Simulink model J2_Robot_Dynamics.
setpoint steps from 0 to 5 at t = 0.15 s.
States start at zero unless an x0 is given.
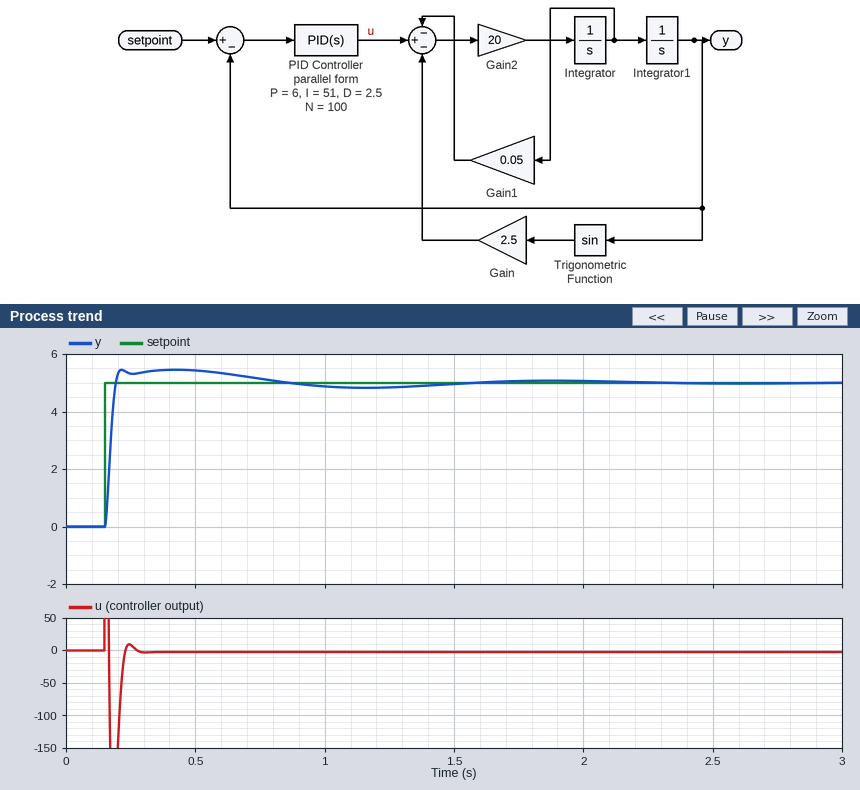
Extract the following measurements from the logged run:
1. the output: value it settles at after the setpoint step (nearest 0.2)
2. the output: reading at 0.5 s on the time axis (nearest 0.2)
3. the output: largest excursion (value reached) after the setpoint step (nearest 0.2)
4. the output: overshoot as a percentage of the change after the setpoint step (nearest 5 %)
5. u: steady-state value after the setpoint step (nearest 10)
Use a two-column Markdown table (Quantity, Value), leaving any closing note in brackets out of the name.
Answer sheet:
| Quantity | Value |
|---|---|
| the output: value it settles at after the setpoint step | 5.0 |
| the output: reading at 0.5 s on the time axis | 5.4 |
| the output: largest excursion (value reached) after the setpoint step | 5.4 |
| the output: overshoot as a percentage of the change after the setpoint step | 10 % |
| u: steady-state value after the setpoint step | 0 |
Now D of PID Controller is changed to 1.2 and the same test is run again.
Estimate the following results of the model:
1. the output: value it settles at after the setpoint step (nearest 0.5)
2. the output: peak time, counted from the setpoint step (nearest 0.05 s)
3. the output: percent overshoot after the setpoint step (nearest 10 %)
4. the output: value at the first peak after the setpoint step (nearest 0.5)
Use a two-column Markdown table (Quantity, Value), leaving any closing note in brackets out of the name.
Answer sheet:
| Quantity | Value |
|---|---|
| the output: value it settles at after the setpoint step | 5.0 |
| the output: peak time, counted from the setpoint step | 0.20 s |
| the output: percent overshoot after the setpoint step | 20 % |
| the output: value at the first peak after the setpoint step | 6.0 |
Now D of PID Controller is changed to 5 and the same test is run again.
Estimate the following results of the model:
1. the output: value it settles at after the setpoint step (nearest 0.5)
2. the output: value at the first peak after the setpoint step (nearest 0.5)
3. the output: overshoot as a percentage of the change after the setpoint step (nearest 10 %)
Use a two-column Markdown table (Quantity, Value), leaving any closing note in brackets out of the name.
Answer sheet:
| Quantity | Value |
|---|---|
| the output: value it settles at after the setpoint step | 5.0 |
| the output: value at the first peak after the setpoint step | 6.0 |
| the output: overshoot as a percentage of the change after the setpoint step | 20 % |
